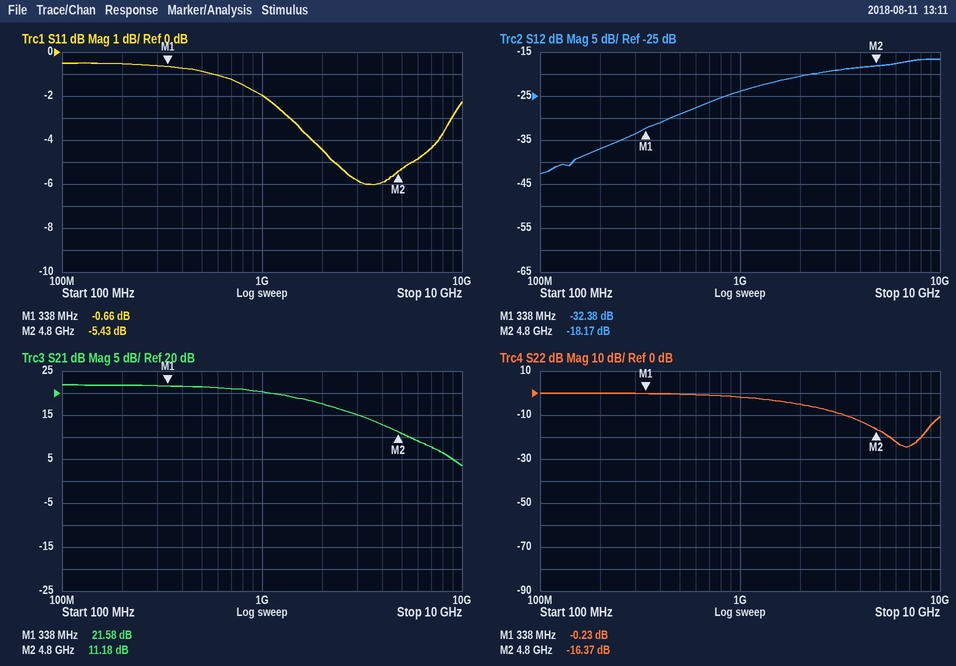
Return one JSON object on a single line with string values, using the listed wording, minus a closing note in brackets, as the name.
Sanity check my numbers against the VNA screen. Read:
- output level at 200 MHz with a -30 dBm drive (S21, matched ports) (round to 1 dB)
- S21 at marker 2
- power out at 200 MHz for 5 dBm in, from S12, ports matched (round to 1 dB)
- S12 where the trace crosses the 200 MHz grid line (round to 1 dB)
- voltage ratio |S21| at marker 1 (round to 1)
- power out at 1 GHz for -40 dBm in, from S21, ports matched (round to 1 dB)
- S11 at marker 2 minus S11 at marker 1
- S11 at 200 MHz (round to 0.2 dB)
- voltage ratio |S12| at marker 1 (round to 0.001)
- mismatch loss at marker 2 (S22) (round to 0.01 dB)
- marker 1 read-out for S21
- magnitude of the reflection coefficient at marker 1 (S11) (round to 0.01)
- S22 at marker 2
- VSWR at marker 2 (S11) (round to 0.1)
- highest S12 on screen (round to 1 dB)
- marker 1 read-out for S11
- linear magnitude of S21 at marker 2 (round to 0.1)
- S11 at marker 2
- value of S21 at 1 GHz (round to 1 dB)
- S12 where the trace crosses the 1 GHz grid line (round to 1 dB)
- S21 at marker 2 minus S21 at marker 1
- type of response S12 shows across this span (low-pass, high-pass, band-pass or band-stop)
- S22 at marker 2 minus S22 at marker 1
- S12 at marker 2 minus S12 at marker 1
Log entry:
{"output level at 200 MHz with a -30 dBm drive (S21, matched ports)": "-8 dBm", "S21 at marker 2": "11.18 dB", "power out at 200 MHz for 5 dBm in, from S12, ports matched": "-32 dBm", "S12 where the trace crosses the 200 MHz grid line": "-37 dB", "voltage ratio |S21| at marker 1": "12", "power out at 1 GHz for -40 dBm in, from S21, ports matched": "-20 dBm", "S11 at marker 2 minus S11 at marker 1": "-4.77 dB", "S11 at 200 MHz": "-0.6 dB", "voltage ratio |S12| at marker 1": "0.024", "mismatch loss at marker 2 (S22)": "0.10 dB", "marker 1 read-out for S21": "21.58 dB", "magnitude of the reflection coefficient at marker 1 (S11)": "0.93", "S22 at marker 2": "-16.37 dB", "VSWR at marker 2 (S11)": "3.3", "highest S12 on screen": "-17 dB", "marker 1 read-out for S11": "-0.66 dB", "linear magnitude of S21 at marker 2": "3.6", "S11 at marker 2": "-5.43 dB", "value of S21 at 1 GHz": "20 dB", "S12 where the trace crosses the 1 GHz grid line": "-24 dB", "S21 at marker 2 minus S21 at marker 1": "-10.40 dB", "type of response S12 shows across this span": "high-pass", "S22 at marker 2 minus S22 at marker 1": "-16.14 dB", "S12 at marker 2 minus S12 at marker 1": "14.21 dB"}
